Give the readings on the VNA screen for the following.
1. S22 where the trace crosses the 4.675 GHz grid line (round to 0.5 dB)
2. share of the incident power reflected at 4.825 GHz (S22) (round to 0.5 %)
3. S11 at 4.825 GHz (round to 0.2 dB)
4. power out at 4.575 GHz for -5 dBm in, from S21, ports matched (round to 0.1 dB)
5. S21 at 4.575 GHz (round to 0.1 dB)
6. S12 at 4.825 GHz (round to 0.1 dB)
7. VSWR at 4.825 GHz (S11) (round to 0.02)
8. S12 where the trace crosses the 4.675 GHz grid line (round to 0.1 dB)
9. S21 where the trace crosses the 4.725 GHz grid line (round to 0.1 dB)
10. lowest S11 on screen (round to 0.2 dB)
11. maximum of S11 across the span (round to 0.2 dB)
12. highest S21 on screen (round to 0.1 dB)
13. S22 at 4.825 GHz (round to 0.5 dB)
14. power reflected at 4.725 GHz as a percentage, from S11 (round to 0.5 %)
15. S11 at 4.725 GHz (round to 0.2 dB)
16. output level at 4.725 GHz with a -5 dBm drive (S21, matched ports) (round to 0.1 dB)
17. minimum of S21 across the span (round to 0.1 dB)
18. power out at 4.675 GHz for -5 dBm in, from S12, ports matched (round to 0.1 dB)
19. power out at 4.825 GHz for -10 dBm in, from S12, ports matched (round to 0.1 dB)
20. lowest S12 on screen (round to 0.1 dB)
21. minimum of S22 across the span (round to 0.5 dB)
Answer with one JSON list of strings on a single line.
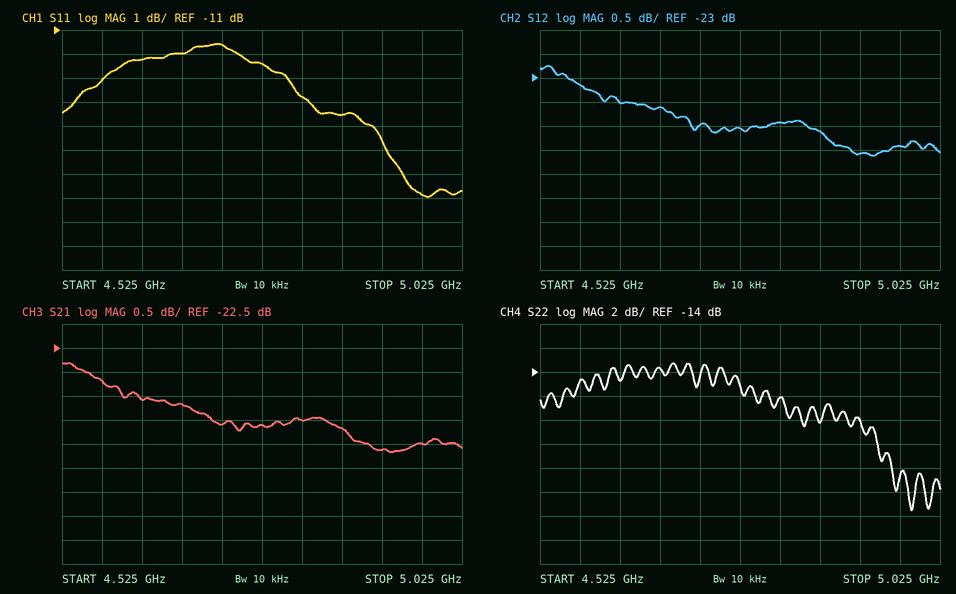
["-13.5 dB", "2.5 %", "-13.8 dB", "-28.2 dBm", "-23.2 dB", "-23.9 dB", "1.52", "-23.6 dB", "-24.1 dB", "-18.0 dB", "-11.6 dB", "-22.8 dB", "-16.0 dB", "7.0 %", "-11.6 dB", "-29.1 dBm", "-24.7 dB", "-28.6 dBm", "-33.9 dBm", "-24.6 dB", "-25.5 dB"]
